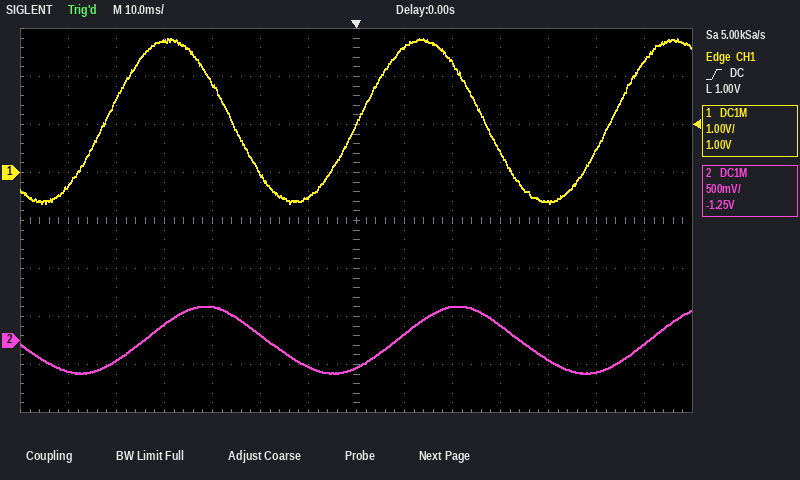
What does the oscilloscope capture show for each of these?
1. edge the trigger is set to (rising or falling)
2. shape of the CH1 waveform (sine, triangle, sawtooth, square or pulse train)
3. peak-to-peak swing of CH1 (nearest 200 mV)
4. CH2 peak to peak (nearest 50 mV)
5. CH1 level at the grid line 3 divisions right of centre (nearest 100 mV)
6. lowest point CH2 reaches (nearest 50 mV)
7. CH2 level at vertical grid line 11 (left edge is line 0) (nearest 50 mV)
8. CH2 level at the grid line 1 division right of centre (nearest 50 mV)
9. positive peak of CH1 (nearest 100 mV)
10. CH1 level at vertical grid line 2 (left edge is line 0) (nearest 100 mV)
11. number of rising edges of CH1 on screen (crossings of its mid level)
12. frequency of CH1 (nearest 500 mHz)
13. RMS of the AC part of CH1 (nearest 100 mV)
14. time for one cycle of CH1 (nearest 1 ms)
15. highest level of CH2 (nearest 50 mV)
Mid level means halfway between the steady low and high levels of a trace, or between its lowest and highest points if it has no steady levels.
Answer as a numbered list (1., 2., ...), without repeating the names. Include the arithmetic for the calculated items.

1. rising
2. sine
3. 3.4 V
4. 350 mV − (-350 mV) = 700 mV
5. 400 mV
6. -350 mV
7. -200 mV
8. 50 mV
9. 2.8 V
10. 1.5 V
11. 3
12. 1 / 53 ms ≈ 18.9 Hz, so 19.0 Hz to the nearest 500 mHz
13. 3.4 V / (2√2) ≈ 1.2 V
14. 53 ms
15. 350 mV
